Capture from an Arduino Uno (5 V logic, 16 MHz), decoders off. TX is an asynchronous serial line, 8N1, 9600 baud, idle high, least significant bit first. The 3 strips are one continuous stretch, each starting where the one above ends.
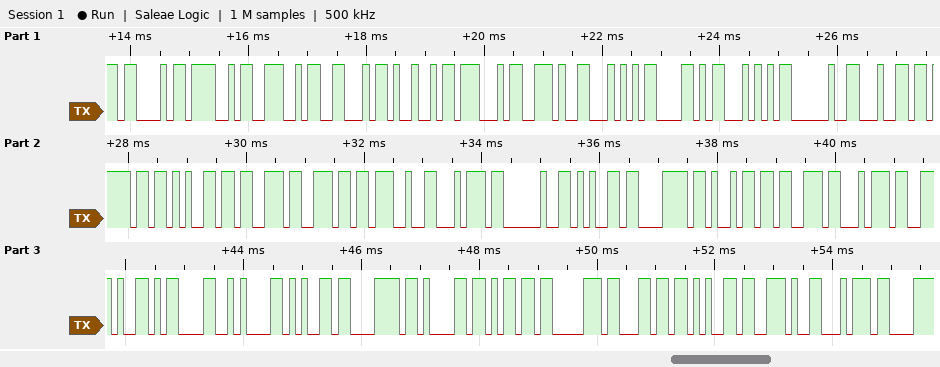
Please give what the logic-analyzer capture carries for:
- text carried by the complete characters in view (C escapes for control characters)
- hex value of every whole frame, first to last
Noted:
"CONFIG.TXT doesn't exist.\r\nexample.t"
0x43 0x4F 0x4E 0x46 0x49 0x47 0x2E 0x54 0x58 0x54 0x20 0x64 0x6F 0x65 0x73 0x6E 0x27 0x74 0x20 0x65 0x78 0x69 0x73 0x74 0x2E 0x0D 0x0A 0x65 0x78 0x61 0x6D 0x70 0x6C 0x65 0x2E 0x74
